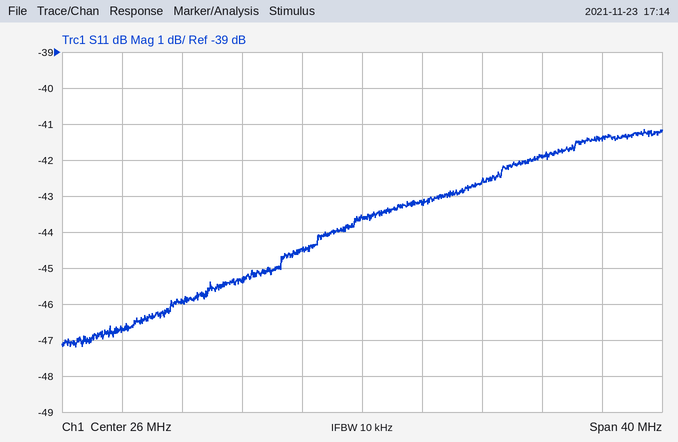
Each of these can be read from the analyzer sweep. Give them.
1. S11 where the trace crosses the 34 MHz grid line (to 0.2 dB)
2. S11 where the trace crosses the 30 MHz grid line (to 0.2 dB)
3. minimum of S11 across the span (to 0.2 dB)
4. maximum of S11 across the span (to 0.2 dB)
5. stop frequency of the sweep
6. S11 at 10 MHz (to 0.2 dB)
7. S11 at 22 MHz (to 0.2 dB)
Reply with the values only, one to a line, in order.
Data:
-42.6 dB
-43.2 dB
-47.2 dB
-41.2 dB
46 MHz
-46.8 dB
-44.4 dB
